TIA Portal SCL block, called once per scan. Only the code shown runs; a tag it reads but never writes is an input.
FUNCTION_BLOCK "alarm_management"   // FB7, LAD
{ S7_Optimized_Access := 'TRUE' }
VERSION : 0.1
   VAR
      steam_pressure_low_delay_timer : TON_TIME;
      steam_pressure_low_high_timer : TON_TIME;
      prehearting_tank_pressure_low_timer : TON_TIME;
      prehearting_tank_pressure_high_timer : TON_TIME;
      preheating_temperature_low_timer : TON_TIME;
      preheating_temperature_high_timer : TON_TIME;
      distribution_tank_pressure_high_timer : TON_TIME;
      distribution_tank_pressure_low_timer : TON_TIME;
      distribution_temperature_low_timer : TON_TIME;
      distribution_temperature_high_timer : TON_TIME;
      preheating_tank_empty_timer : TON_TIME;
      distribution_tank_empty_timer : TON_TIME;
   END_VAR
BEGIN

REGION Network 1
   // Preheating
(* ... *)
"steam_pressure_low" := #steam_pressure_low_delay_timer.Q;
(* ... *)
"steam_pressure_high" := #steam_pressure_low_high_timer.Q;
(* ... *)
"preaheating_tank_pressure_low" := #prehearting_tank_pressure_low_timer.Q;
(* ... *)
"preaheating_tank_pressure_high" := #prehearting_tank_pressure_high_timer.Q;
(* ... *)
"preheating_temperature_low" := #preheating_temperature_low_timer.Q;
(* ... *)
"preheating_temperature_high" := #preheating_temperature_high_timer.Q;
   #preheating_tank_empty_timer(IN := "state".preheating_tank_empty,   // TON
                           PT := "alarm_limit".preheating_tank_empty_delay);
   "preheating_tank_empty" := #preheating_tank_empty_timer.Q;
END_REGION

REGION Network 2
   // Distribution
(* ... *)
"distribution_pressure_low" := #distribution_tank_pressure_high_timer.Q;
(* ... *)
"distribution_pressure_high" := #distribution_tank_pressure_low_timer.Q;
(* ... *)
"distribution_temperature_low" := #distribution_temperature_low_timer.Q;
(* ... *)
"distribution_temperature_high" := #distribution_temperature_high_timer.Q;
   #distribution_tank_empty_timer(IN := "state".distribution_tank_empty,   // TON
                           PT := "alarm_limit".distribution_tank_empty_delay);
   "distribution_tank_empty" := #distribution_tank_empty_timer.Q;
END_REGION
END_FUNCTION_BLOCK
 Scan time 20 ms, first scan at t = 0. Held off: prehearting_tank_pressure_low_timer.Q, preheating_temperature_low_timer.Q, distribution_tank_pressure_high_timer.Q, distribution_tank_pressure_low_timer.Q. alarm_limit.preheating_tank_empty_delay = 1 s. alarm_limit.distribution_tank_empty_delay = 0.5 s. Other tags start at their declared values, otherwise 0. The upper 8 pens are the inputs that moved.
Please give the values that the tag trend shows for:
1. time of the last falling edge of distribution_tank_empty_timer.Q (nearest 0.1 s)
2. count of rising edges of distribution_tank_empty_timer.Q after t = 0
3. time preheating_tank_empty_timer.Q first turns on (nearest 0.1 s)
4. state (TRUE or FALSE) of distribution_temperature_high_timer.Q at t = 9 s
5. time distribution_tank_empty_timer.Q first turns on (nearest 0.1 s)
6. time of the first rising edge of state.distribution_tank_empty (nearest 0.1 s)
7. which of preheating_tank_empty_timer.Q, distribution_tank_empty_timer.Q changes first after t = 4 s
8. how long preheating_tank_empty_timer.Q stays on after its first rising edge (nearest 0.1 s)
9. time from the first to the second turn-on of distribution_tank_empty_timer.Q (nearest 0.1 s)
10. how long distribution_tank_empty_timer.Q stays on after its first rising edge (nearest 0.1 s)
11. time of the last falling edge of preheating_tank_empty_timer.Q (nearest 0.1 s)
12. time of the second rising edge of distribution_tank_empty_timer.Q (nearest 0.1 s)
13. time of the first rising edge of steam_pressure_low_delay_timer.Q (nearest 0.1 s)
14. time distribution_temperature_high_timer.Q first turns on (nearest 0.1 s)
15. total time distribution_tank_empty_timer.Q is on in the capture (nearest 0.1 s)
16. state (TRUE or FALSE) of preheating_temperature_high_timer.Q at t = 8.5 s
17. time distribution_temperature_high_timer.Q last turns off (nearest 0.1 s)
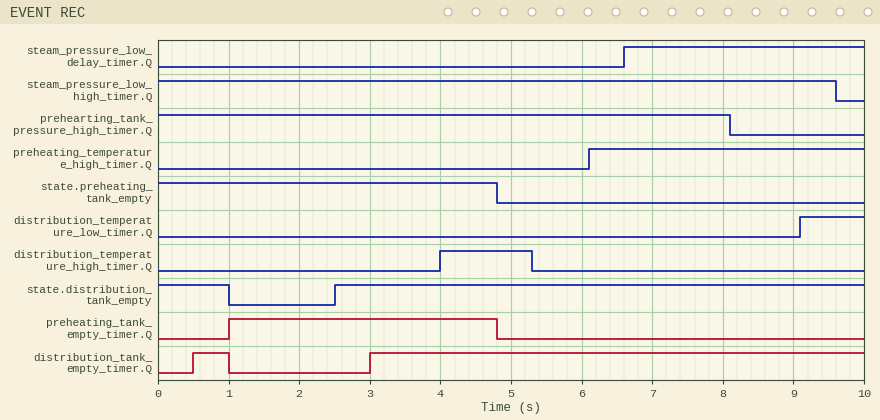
1.0 s
2
1.0 s
FALSE
0.5 s
2.5 s
preheating_tank_empty_timer.Q
3.8 s
2.5 s
0.5 s
4.8 s
3.0 s
6.6 s
4.0 s
7.5 s
TRUE
5.3 s
